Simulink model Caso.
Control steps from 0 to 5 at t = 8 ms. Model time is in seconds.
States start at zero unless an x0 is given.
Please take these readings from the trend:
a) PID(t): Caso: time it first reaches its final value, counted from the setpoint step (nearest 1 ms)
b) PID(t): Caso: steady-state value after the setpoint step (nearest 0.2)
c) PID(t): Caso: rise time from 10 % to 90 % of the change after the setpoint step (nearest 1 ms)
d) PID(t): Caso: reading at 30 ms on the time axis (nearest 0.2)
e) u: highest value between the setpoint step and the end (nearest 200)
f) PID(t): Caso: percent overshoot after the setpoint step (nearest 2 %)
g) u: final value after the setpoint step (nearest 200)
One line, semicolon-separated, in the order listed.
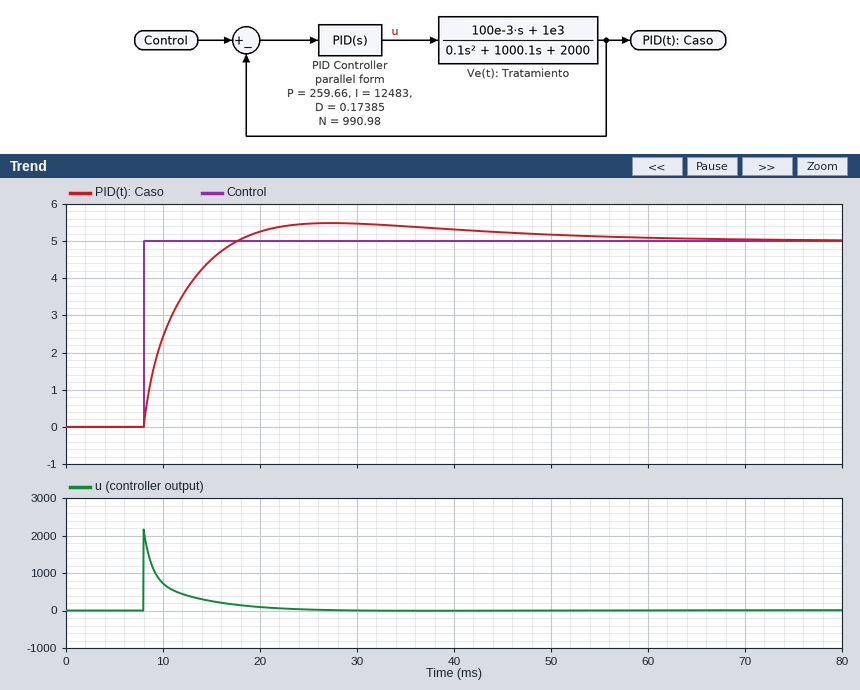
10 ms; 5.0; 7 ms; 5.4; 2200; 10 %; 0
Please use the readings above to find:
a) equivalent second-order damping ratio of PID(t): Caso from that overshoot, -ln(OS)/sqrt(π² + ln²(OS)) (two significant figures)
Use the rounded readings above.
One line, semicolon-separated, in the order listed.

0.59
